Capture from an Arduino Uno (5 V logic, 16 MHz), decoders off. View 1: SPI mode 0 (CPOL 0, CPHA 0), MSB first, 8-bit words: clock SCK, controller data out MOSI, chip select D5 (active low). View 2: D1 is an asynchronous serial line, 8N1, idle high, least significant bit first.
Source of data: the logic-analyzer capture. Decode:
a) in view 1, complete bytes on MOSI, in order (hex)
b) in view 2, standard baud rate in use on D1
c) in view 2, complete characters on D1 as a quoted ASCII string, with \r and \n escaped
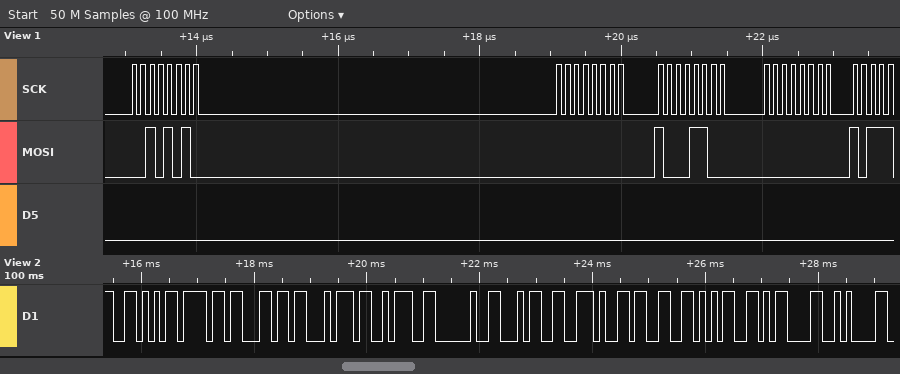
0x2A 0x00 0x8C 0x00
9600 baud
"Volt: 4.35\r\n"
